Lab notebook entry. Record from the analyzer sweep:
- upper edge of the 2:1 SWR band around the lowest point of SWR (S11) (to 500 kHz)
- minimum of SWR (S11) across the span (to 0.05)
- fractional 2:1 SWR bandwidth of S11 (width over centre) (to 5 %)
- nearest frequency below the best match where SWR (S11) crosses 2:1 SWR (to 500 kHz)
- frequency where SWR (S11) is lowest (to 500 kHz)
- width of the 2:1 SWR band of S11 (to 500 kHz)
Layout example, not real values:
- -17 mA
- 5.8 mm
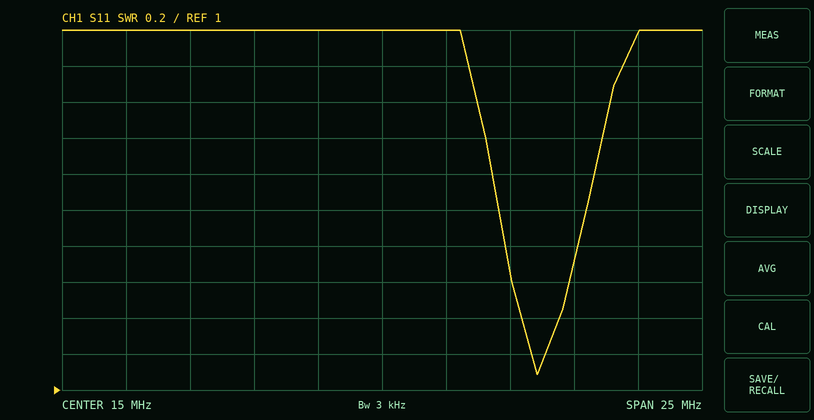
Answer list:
- 23.0 MHz
- 1.10
- 15 %
- 19.5 MHz
- 21.0 MHz
- 3.5 MHz
